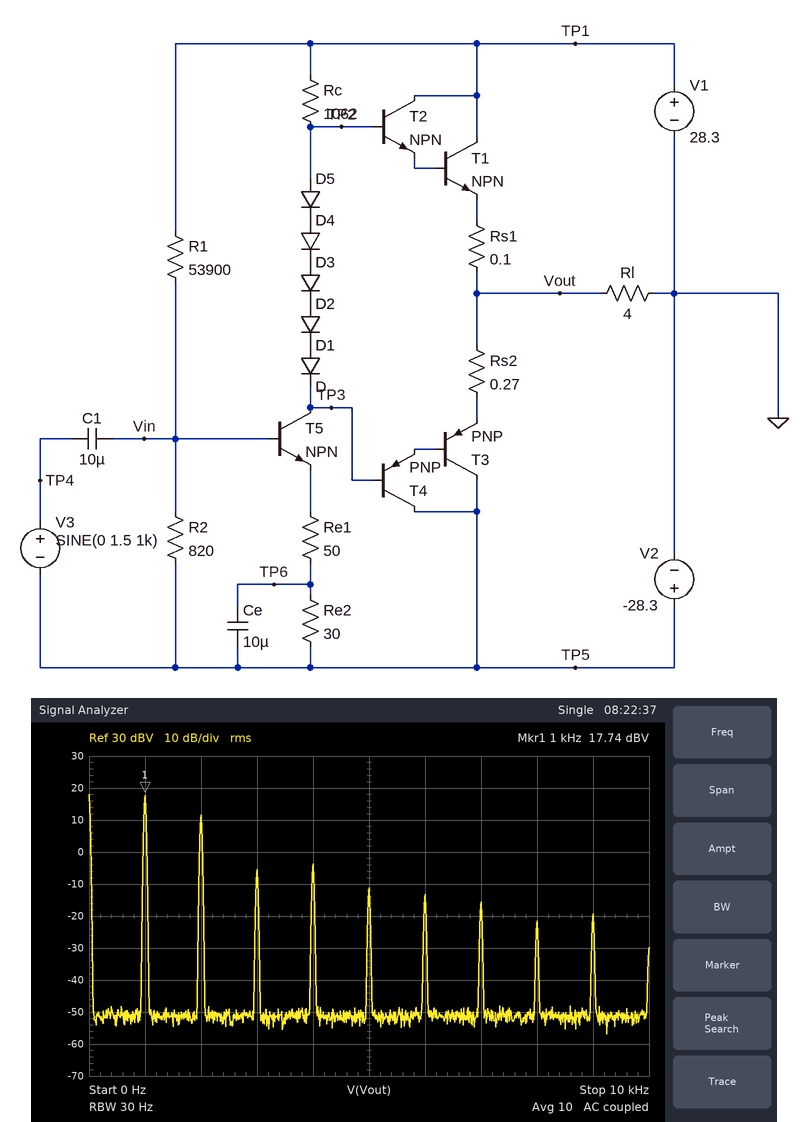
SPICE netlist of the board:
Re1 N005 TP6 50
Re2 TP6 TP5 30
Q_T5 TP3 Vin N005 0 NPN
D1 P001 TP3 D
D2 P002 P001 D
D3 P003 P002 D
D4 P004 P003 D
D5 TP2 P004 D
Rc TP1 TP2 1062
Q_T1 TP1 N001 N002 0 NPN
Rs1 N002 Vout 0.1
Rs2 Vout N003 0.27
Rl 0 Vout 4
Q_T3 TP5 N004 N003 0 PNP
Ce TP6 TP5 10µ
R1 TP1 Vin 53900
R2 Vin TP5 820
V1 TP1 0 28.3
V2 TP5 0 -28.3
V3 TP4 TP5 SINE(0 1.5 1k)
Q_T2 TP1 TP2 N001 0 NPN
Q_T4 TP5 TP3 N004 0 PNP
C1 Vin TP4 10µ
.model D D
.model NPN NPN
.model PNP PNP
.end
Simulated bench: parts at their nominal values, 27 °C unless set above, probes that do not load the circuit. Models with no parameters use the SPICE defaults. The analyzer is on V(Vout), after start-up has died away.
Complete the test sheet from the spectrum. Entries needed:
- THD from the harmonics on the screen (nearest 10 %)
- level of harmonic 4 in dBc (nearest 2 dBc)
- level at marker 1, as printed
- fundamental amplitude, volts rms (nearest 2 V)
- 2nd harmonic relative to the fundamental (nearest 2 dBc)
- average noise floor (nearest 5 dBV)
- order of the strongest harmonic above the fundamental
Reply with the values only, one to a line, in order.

50 %
-22 dBc
17.74 dBV
8 V
-6 dBc
-50 dBV
2
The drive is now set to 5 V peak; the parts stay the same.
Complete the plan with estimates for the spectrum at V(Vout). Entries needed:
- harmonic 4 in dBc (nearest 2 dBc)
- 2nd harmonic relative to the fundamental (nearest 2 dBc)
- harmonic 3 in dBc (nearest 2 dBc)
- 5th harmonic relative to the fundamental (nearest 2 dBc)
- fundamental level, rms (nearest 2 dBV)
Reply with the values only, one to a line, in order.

-18 dBc
-4 dBc
-18 dBc
-16 dBc
24 dBV
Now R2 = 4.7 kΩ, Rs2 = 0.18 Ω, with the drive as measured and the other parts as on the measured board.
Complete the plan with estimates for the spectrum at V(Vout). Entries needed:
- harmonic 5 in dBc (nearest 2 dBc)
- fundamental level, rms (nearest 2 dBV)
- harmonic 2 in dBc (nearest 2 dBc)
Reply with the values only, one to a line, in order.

-38 dBc
24 dBV
-48 dBc
